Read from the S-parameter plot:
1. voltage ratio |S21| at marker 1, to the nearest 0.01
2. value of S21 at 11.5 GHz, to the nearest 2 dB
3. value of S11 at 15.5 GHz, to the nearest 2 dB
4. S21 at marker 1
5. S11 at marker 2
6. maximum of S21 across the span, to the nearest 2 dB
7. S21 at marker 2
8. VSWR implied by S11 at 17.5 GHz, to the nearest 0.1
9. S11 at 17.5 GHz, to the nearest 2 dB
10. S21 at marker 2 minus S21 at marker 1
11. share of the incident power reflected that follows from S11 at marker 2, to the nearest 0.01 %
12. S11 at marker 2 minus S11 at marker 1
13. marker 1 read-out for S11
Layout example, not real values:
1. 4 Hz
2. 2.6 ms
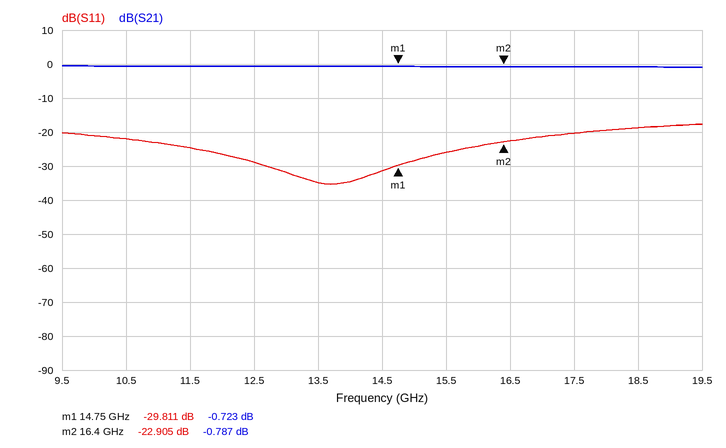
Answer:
1. 0.92
2. 0 dB
3. -26 dB
4. -0.723 dB
5. -22.905 dB
6. 0 dB
7. -0.787 dB
8. 1.2
9. -20 dB
10. -0.064 dB
11. 0.51 %
12. 6.906 dB
13. -29.811 dB
